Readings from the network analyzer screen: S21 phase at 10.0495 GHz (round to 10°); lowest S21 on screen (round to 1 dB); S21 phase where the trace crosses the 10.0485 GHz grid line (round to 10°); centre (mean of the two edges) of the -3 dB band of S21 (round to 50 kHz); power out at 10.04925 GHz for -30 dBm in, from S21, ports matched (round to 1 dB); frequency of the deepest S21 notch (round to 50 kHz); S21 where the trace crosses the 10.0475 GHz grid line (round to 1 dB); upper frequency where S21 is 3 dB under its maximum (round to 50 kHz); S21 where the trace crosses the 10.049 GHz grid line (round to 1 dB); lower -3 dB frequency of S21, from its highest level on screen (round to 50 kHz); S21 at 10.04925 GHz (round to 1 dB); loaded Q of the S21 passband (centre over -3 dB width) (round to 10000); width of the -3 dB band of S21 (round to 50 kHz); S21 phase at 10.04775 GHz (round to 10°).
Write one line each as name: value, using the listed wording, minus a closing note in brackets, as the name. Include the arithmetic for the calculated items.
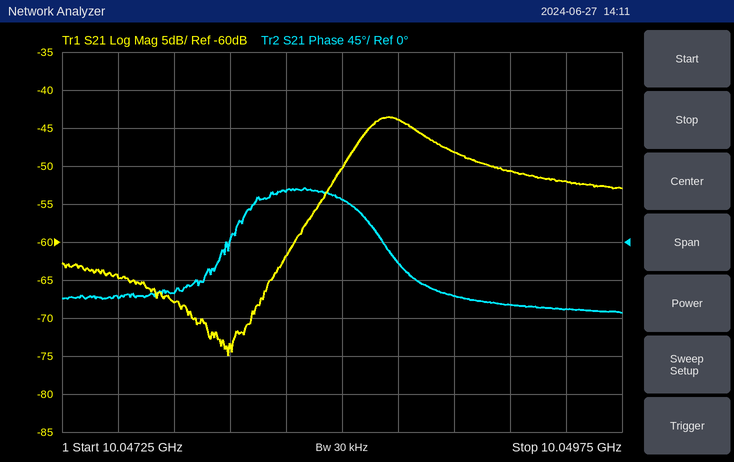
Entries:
S21 phase at 10.0495 GHz: -80°
lowest S21 on screen: -75 dB
S21 phase where the trace crosses the 10.0485 GHz grid line: 50°
centre (mean of the two edges) of the -3 dB band of S21: 10.04875 GHz
power out at 10.04925 GHz for -30 dBm in, from S21, ports matched: -30 dBm + (-51 dB) = -81 dBm
frequency of the deepest S21 notch: 10.04800 GHz
S21 where the trace crosses the 10.0475 GHz grid line: -65 dB
upper frequency where S21 is 3 dB under its maximum: 10.04890 GHz
S21 where the trace crosses the 10.049 GHz grid line: -48 dB
lower -3 dB frequency of S21, from its highest level on screen: 10.04860 GHz
S21 at 10.04925 GHz: -51 dB
loaded Q of the S21 passband (centre over -3 dB width): 10.0488 GHz / 300 kHz ≈ 33496, so 30000 to the nearest 10000
width of the -3 dB band of S21: 10.04890 GHz − 10.04860 GHz = 300 kHz
S21 phase at 10.04775 GHz: -60°
